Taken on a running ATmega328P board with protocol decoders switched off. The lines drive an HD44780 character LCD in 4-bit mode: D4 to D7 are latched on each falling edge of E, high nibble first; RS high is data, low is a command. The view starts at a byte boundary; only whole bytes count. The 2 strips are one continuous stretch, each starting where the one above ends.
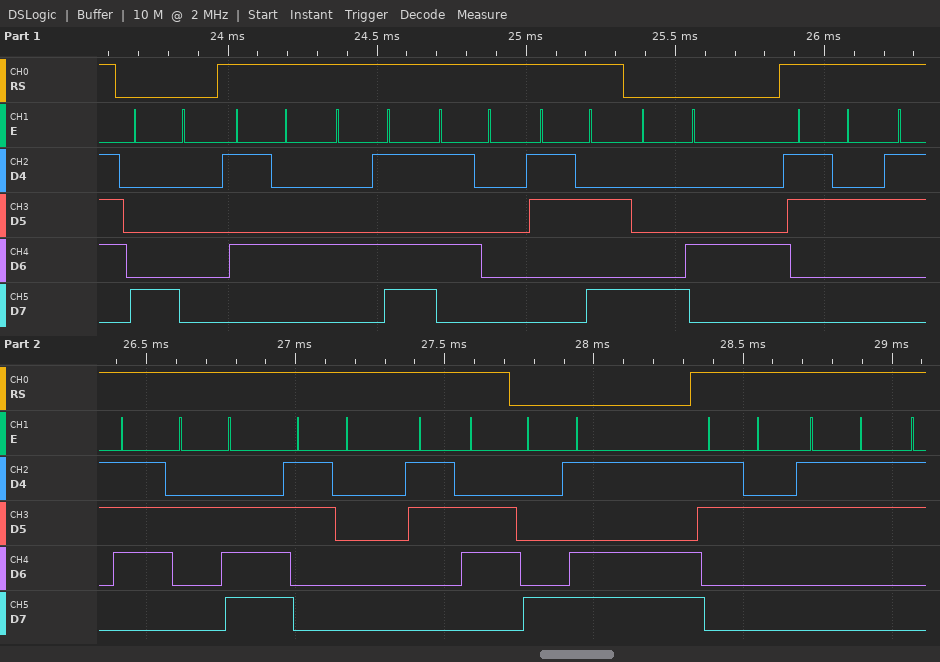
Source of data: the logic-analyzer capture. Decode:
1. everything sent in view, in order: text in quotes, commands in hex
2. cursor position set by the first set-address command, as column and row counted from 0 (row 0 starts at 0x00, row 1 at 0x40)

0x80 "TMP:" 0x84 "27.06" 0x8D "23"
column 0, row 0
